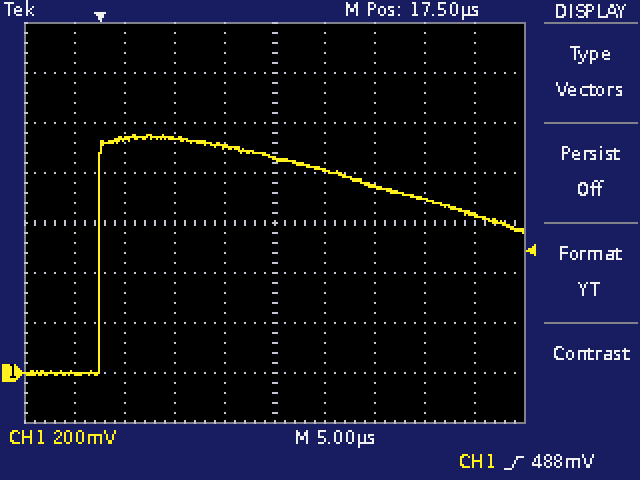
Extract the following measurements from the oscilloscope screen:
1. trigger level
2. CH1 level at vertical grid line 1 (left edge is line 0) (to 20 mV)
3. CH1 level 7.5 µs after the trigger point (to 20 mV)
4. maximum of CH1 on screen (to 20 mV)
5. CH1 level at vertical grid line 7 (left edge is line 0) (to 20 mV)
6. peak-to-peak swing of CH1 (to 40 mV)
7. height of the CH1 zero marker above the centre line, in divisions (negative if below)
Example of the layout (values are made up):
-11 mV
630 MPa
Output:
488 mV
0 mV
940 mV
960 mV
740 mV
960 mV
-3.0 div
